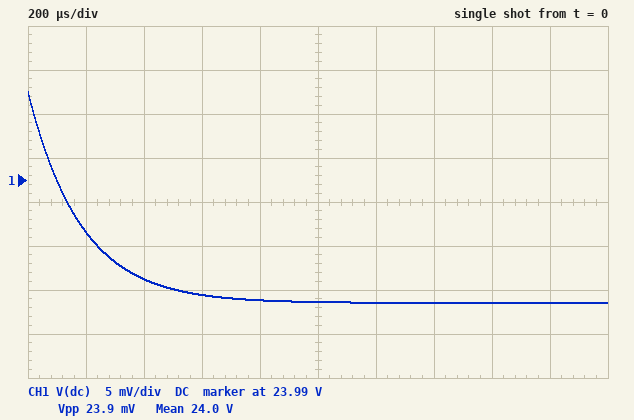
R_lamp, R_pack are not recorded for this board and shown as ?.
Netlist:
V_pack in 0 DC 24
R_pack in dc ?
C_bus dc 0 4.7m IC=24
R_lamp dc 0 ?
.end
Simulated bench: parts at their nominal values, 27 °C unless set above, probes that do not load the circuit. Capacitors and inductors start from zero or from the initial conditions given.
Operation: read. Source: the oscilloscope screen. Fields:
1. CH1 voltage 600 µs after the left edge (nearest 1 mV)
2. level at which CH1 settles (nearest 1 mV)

23.977 V
23.976 V
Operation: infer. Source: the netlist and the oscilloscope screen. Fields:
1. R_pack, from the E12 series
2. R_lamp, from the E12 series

0.039 Ω
39 Ω
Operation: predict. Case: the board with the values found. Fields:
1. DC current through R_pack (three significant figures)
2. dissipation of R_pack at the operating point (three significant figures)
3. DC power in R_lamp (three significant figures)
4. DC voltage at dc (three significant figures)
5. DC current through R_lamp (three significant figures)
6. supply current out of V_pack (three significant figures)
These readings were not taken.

615 mA
14.7 mW
14.7 W
24.0 V
615 mA
615 mA
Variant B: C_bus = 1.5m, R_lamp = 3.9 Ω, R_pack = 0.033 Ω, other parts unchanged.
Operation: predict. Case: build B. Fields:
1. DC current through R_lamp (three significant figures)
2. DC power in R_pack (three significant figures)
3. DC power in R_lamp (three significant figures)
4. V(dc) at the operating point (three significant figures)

6.10 A
1.23 W
145 W
23.8 V
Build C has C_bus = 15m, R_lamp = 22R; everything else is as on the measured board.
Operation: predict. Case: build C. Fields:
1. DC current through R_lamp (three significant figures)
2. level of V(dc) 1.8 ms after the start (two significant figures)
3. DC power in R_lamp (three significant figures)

1.09 A
24 V
26.1 W
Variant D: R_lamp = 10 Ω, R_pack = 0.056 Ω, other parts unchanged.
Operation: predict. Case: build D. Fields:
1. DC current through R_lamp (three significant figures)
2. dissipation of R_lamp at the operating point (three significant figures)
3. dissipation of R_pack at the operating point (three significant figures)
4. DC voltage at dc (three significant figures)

2.39 A
57.0 W
319 mW
23.9 V
